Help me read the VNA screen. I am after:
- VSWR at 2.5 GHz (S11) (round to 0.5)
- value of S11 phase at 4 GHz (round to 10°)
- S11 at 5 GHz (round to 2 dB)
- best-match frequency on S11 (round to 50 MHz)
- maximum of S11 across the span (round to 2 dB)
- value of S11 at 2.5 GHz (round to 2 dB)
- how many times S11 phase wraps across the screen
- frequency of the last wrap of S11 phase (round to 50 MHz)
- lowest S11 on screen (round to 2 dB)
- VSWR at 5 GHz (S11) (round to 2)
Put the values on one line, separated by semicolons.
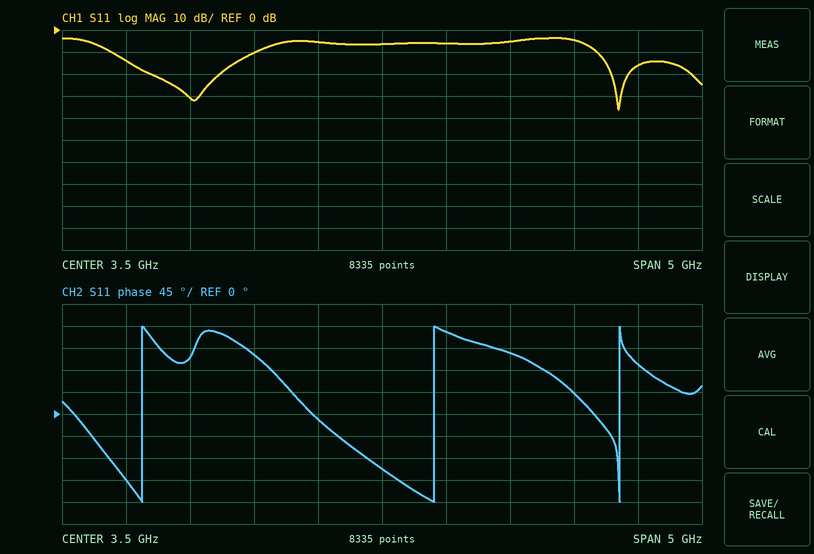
2.0; 170°; -4 dB; 5.35 GHz; -4 dB; -10 dB; 3; 5.35 GHz; -36 dB; 4
